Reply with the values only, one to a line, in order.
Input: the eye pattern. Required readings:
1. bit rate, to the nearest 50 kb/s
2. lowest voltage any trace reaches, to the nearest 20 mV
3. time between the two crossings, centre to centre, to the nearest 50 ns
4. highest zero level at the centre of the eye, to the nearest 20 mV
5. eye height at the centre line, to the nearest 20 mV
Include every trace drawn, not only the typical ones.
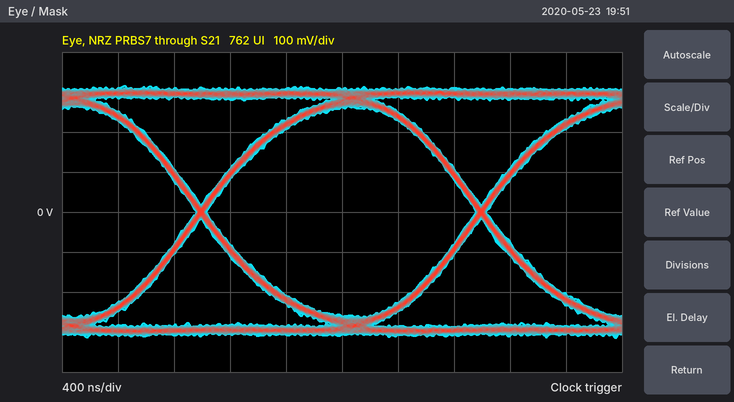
500 kb/s
-320 mV
2.00 µs
-260 mV
520 mV
